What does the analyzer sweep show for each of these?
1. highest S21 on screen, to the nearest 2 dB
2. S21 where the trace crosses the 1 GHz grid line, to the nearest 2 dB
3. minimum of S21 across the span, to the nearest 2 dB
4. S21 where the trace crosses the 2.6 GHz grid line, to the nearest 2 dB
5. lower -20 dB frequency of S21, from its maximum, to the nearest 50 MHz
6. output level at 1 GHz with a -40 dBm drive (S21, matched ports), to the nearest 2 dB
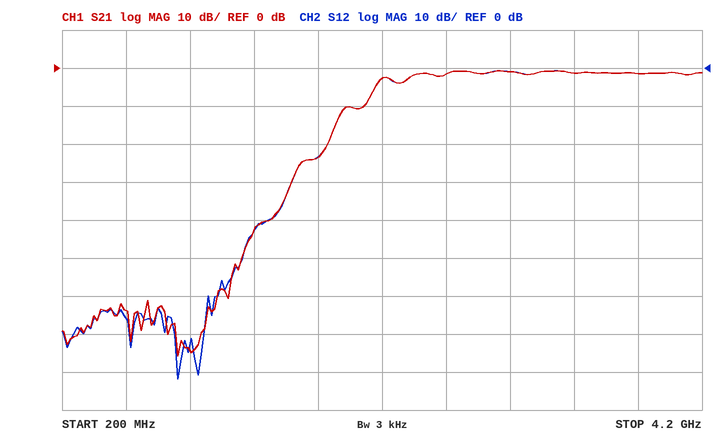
0 dB
-74 dB
-76 dB
-2 dB
1.85 GHz
-114 dBm
